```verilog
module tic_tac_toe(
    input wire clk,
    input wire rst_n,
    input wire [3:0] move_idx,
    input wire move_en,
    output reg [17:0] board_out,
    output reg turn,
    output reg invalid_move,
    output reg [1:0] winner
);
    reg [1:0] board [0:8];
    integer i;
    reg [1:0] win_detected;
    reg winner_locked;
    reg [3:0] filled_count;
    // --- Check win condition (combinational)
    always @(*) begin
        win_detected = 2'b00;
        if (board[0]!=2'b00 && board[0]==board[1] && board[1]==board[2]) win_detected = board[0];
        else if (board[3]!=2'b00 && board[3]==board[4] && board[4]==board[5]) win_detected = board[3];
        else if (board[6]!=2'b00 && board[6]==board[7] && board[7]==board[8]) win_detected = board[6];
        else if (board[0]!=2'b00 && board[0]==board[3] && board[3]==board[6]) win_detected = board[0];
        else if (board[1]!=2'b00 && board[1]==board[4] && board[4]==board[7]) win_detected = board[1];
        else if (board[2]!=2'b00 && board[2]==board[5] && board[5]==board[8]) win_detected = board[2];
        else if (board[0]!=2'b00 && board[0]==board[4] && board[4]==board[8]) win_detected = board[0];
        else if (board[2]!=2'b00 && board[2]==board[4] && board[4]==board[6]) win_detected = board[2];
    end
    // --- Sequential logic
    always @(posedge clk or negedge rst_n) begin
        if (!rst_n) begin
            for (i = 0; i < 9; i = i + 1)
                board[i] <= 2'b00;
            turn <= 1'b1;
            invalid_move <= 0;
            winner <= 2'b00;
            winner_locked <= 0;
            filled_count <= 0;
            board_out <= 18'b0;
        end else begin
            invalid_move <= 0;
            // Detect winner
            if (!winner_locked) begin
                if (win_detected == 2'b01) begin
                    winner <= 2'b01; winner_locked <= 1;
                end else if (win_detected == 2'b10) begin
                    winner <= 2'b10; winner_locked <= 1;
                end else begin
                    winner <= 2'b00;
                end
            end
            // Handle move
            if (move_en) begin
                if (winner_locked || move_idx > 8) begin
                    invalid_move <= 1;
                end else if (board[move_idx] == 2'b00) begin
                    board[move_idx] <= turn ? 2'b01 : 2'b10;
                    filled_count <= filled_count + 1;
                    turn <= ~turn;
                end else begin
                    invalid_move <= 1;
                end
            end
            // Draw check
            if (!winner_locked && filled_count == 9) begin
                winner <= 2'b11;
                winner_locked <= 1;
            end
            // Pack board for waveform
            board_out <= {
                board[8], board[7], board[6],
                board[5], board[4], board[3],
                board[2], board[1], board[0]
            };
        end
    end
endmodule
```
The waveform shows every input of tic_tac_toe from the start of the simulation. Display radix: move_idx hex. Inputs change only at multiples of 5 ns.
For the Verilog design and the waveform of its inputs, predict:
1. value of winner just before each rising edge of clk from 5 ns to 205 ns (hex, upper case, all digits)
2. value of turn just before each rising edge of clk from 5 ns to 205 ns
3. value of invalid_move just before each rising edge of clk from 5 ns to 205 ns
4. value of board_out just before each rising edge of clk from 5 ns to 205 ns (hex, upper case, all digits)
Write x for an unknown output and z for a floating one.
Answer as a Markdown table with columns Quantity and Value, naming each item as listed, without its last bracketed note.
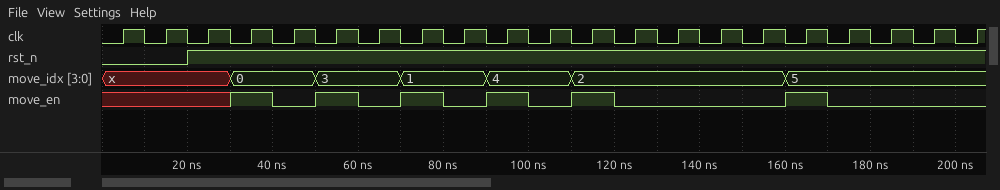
| Quantity | Value |
|---|---|
| value of winner just before each rising edge of clk from 5 ns to 205 ns | 0, 0, 0, 0, 0, 0, 0, 0, 0, 0, 0, 0, 0, 1, 1, 1, 1, 1, 1, 1, 1 |
| value of turn just before each rising edge of clk from 5 ns to 205 ns | 1 1 1 1 0 0 1 1 0 0 1 1 0 0 0 0 0 0 0 0 0 |
| value of invalid_move just before each rising edge of clk from 5 ns to 205 ns | 0 0 0 0 0 0 0 0 0 0 0 0 0 0 0 0 0 1 0 0 0 |
| value of board_out just before each rising edge of clk from 5 ns to 205 ns | 00000, 00000, 00000, 00000, 00000, 00001, 00001, 00081, 00081, 00085, 00085, 00285, 00285, 00295, 00295, 00295, 00295, 00295, 00295, 00295, 00295 |
